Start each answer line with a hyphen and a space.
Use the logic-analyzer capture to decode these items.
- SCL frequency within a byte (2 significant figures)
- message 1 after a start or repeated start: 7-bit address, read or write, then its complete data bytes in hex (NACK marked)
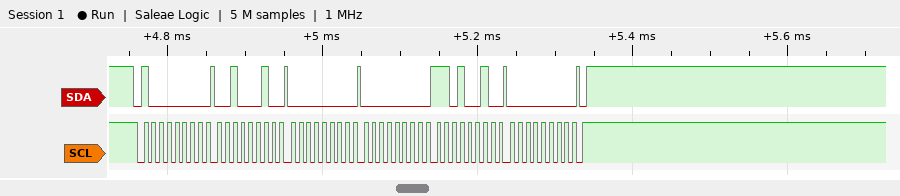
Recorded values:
- 100 kHz
- 0x40 write: 22 00 00 D2 00
